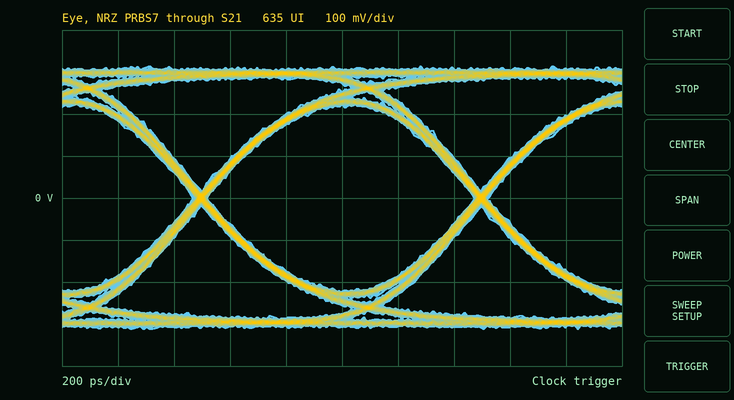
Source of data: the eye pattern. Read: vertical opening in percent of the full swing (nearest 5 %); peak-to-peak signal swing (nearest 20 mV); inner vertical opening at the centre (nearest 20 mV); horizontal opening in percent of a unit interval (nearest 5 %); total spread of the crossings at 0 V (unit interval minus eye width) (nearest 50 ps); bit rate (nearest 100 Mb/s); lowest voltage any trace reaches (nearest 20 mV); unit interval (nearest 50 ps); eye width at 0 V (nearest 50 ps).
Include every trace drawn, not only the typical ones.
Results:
70 %
620 mV
440 mV
95 %
50 ps
1.0 Gb/s
-320 mV
1.00 ns
950 ps
